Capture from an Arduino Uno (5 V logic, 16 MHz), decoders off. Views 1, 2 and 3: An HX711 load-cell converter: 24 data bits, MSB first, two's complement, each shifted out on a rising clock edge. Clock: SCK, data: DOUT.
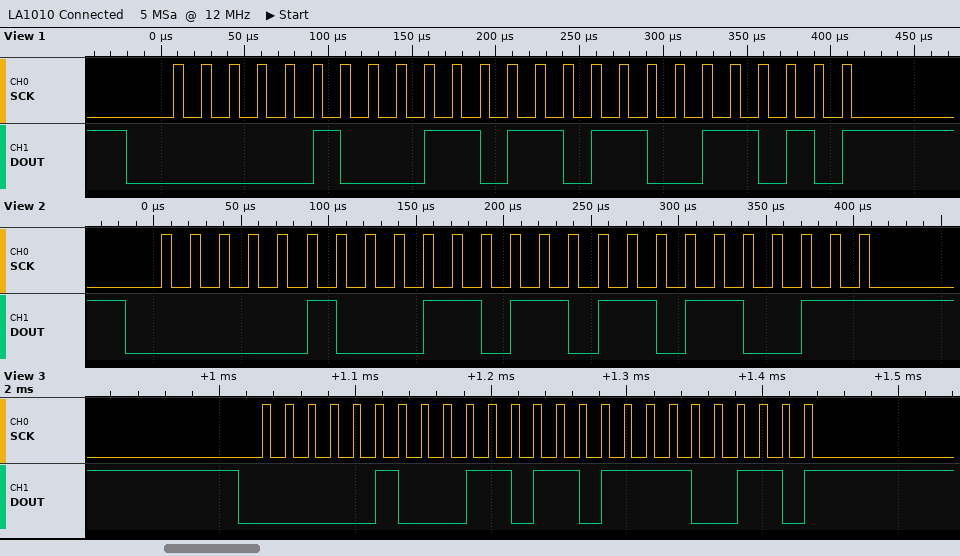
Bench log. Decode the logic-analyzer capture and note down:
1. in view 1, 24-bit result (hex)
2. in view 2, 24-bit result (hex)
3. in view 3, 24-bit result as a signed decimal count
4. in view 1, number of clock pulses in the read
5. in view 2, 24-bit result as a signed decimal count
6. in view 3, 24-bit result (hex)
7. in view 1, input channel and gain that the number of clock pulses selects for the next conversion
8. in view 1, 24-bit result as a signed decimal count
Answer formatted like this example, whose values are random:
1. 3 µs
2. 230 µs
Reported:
1. 0x046D9A
2. 0x046DB3
3. 290278
4. 25
5. 290227
6. 0x046DE6
7. channel A, gain 128
8. 290202
